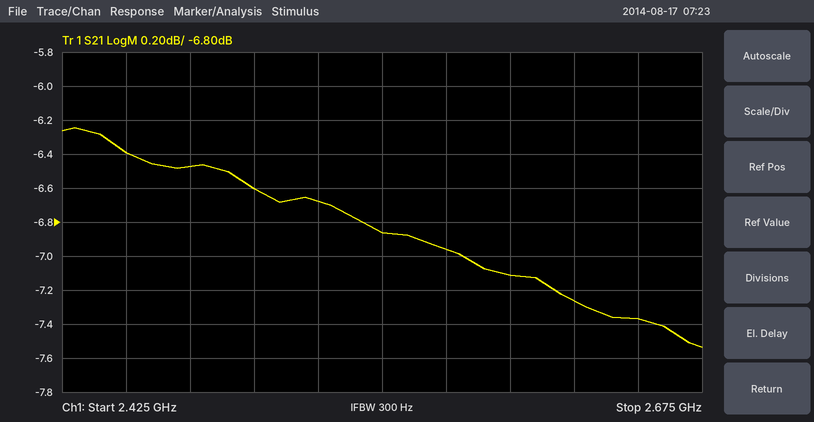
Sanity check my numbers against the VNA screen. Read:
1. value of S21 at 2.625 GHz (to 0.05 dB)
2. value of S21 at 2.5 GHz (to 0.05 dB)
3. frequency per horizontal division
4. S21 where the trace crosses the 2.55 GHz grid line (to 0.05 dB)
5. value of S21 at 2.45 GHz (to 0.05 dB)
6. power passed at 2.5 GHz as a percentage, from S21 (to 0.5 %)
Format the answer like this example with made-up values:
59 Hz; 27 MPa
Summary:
-7.25 dB; -6.60 dB; 25 MHz; -6.85 dB; -6.40 dB; 22.0 %
